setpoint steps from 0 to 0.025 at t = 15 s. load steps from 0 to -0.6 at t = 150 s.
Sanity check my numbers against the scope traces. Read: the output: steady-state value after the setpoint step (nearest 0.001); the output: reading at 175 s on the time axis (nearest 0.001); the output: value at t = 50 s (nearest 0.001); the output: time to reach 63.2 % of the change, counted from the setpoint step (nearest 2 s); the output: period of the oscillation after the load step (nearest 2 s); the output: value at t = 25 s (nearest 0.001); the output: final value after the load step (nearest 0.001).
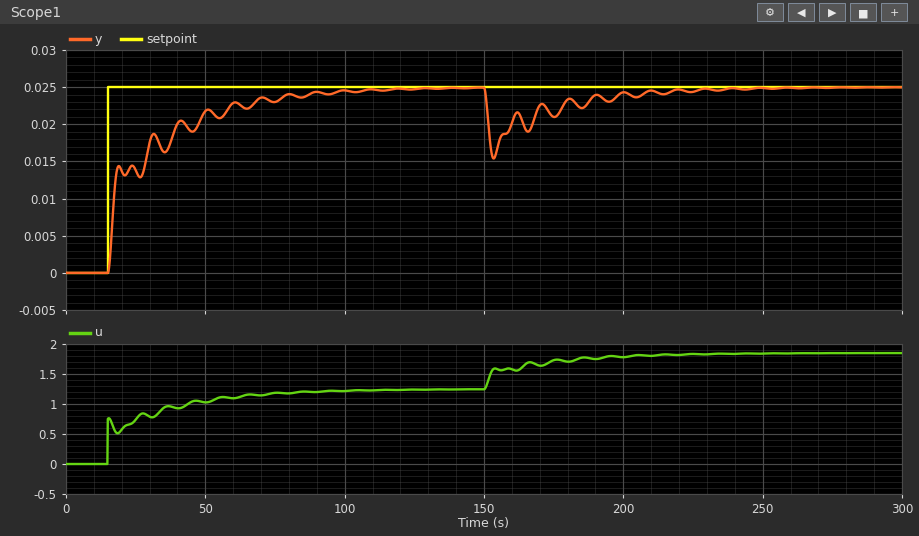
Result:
0.025
0.021
0.022
14 s
12 s
0.014
0.025
